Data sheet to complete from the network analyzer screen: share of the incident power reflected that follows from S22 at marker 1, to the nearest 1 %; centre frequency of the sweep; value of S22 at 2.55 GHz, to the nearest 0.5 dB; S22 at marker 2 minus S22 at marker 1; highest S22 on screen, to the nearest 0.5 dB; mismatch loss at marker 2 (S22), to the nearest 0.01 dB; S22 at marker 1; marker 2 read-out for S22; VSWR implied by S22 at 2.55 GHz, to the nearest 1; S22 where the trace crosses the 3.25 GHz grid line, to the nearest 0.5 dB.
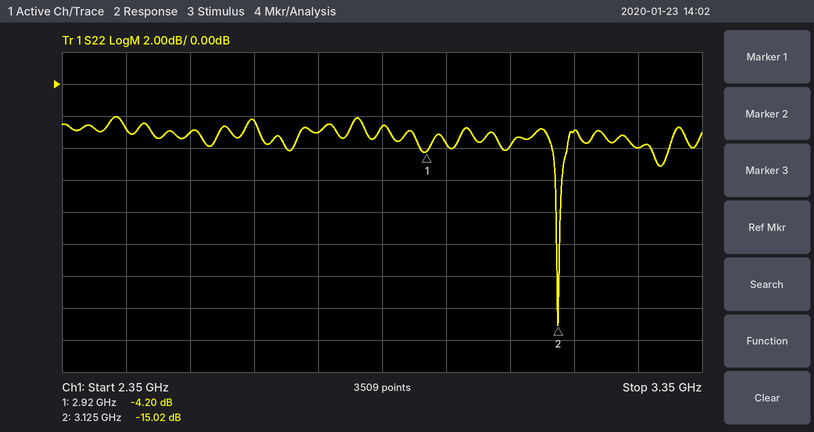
38 %
2.85 GHz
-3.0 dB
-10.82 dB
-2.0 dB
0.14 dB
-4.20 dB
-15.02 dB
6
-4.0 dB
